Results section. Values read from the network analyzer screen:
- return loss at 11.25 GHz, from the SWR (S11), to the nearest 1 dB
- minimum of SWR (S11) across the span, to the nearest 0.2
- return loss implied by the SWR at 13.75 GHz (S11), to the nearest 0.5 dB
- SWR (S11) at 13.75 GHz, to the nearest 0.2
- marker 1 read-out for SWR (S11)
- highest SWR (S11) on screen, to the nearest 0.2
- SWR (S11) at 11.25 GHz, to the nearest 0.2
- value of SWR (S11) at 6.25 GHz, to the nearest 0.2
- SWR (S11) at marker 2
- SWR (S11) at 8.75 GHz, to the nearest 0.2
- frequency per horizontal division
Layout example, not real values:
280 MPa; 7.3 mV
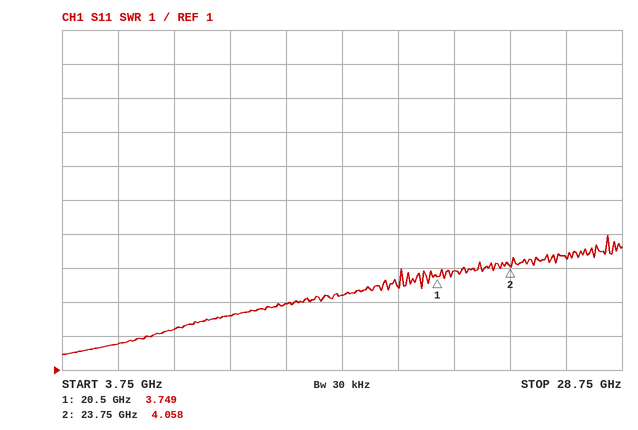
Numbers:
7 dB; 1.4; 6.0 dB; 3.0; 3.749; 5.0; 2.6; 1.8; 4.058; 2.2; 2.5 GHz
